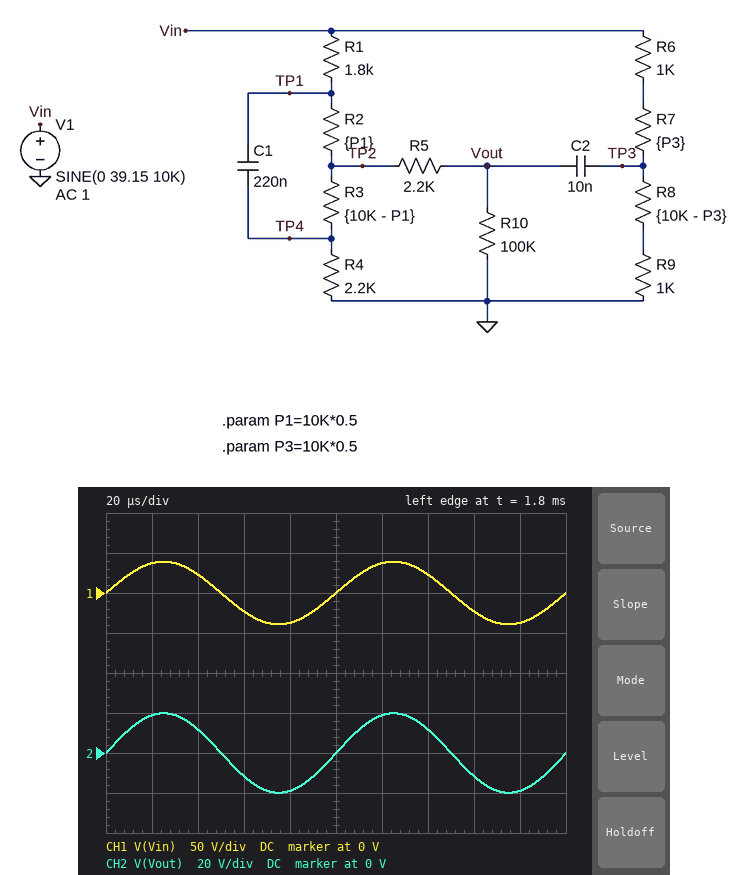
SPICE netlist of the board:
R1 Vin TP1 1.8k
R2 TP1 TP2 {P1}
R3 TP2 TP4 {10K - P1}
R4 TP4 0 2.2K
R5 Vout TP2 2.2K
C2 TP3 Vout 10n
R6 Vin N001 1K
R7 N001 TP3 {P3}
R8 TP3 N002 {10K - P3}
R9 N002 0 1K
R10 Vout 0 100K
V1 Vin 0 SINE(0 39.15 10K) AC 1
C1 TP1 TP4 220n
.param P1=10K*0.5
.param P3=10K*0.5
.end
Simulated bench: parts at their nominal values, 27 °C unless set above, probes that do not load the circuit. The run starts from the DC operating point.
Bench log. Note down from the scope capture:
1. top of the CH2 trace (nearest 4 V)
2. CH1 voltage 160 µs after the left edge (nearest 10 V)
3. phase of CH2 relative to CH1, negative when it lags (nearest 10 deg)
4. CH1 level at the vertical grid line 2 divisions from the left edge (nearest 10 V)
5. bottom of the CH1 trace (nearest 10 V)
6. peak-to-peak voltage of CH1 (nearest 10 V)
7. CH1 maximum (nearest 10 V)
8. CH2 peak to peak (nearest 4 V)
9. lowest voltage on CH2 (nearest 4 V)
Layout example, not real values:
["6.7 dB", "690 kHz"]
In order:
["20 V", "-20 V", "0 deg", "20 V", "-40 V", "80 V", "40 V", "40 V", "-20 V"]
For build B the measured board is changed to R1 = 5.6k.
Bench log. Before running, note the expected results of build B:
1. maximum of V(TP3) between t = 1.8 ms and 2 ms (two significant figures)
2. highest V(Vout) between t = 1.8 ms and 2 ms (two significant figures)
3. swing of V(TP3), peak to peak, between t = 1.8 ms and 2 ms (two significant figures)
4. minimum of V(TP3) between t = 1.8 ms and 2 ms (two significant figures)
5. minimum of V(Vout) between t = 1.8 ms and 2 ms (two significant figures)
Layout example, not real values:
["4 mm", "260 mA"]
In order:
["17 V", "16 V", "33 V", "-17 V", "-16 V"]
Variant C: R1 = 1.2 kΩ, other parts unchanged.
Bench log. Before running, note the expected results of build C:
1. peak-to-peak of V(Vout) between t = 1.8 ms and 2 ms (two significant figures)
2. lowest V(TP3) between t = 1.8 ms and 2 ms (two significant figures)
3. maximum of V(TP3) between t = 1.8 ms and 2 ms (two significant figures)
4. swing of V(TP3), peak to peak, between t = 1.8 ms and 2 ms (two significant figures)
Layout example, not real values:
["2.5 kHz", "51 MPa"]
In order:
["43 V", "-21 V", "21 V", "42 V"]
